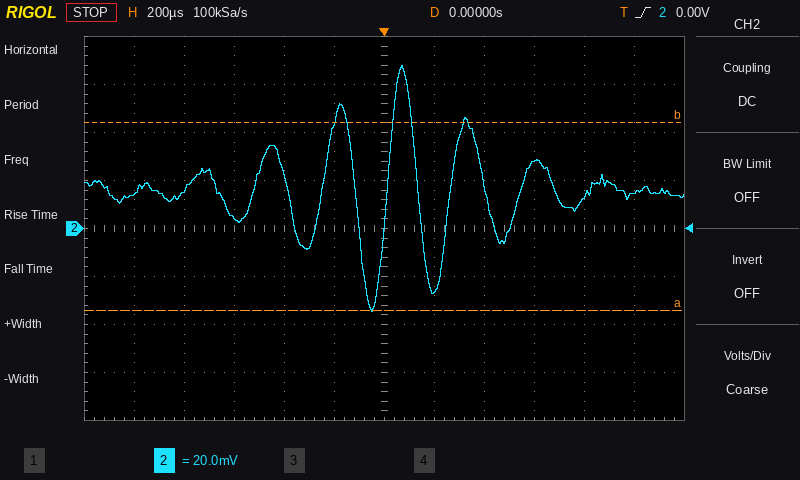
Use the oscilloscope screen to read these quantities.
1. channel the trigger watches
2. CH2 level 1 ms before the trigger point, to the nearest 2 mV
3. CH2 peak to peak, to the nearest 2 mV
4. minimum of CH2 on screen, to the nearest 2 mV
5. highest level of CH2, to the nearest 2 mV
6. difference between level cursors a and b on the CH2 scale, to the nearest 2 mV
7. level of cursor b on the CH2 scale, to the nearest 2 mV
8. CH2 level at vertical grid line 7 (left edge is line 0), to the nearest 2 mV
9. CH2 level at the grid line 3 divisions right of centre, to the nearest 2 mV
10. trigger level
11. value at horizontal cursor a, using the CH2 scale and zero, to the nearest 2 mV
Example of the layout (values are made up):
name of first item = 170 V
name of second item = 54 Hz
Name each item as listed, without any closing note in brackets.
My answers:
channel the trigger watches = CH2
CH2 level 1 ms before the trigger point, to the nearest 2 mV = 14 mV
CH2 peak to peak, to the nearest 2 mV = 102 mV
minimum of CH2 on screen, to the nearest 2 mV = -34 mV
highest level of CH2, to the nearest 2 mV = 68 mV
difference between level cursors a and b on the CH2 scale, to the nearest 2 mV = 78 mV
level of cursor b on the CH2 scale, to the nearest 2 mV = 44 mV
CH2 level at vertical grid line 7 (left edge is line 0), to the nearest 2 mV = -26 mV
CH2 level at the grid line 3 divisions right of centre, to the nearest 2 mV = 28 mV
trigger level = 0.00 V
value at horizontal cursor a, using the CH2 scale and zero, to the nearest 2 mV = -34 mV
